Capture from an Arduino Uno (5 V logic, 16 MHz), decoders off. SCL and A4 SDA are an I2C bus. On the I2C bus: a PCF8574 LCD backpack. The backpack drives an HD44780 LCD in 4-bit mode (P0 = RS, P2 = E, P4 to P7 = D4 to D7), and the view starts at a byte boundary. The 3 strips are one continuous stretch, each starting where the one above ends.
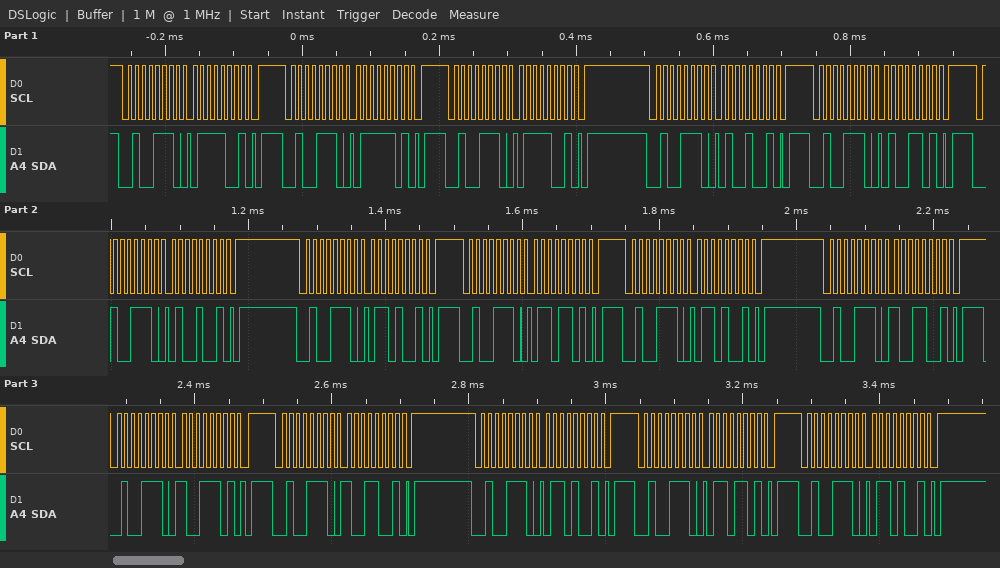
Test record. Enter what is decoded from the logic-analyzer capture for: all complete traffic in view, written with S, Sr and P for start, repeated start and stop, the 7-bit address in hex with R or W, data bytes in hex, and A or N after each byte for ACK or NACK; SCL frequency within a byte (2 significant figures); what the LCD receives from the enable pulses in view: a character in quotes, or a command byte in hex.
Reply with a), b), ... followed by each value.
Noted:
a) S 27W A 79 A P S 27W A 7D A P S 27W A 79 A P S 27W A 49 A P S 27W A 4D A P S 27W A 49 A P S 27W A 69 A P S 27W A 6D A P S 27W A 69 A P S 27W A 99 A P S 27W A 9D A P S 27W A 99 A P S 27W A 69 A P S 27W A 6D A P S 27W A 69 A P
b) 100 kHz
c) 't' 'i'
